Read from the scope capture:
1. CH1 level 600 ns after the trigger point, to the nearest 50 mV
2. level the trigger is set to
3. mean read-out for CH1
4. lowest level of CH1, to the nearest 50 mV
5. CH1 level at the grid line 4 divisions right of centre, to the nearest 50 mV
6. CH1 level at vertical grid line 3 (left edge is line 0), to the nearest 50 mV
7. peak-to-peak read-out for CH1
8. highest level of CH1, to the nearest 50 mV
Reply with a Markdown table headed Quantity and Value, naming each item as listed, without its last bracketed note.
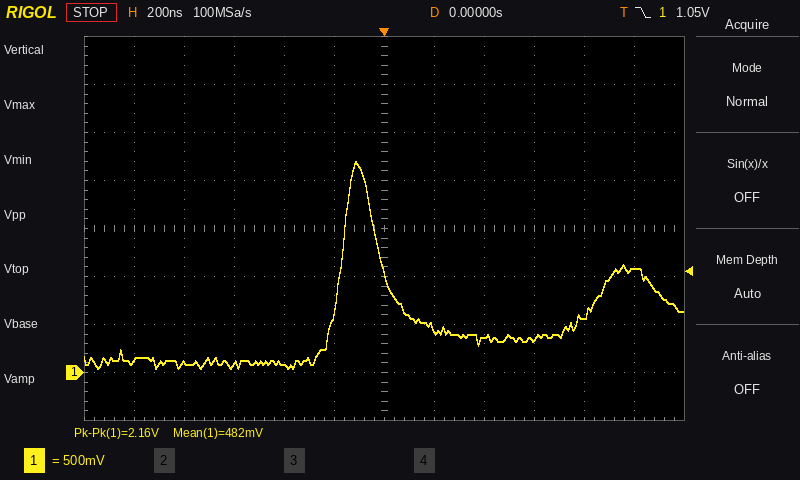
| Quantity | Value |
|---|---|
| CH1 level 600 ns after the trigger point, to the nearest 50 mV | 350 mV |
| level the trigger is set to | 1.05 V |
| mean read-out for CH1 | 482 mV |
| lowest level of CH1, to the nearest 50 mV | 50 mV |
| CH1 level at the grid line 4 divisions right of centre, to the nearest 50 mV | 600 mV |
| CH1 level at vertical grid line 3 (left edge is line 0), to the nearest 50 mV | 100 mV |
| peak-to-peak read-out for CH1 | 2.16 V |
| highest level of CH1, to the nearest 50 mV | 2.20 V |
